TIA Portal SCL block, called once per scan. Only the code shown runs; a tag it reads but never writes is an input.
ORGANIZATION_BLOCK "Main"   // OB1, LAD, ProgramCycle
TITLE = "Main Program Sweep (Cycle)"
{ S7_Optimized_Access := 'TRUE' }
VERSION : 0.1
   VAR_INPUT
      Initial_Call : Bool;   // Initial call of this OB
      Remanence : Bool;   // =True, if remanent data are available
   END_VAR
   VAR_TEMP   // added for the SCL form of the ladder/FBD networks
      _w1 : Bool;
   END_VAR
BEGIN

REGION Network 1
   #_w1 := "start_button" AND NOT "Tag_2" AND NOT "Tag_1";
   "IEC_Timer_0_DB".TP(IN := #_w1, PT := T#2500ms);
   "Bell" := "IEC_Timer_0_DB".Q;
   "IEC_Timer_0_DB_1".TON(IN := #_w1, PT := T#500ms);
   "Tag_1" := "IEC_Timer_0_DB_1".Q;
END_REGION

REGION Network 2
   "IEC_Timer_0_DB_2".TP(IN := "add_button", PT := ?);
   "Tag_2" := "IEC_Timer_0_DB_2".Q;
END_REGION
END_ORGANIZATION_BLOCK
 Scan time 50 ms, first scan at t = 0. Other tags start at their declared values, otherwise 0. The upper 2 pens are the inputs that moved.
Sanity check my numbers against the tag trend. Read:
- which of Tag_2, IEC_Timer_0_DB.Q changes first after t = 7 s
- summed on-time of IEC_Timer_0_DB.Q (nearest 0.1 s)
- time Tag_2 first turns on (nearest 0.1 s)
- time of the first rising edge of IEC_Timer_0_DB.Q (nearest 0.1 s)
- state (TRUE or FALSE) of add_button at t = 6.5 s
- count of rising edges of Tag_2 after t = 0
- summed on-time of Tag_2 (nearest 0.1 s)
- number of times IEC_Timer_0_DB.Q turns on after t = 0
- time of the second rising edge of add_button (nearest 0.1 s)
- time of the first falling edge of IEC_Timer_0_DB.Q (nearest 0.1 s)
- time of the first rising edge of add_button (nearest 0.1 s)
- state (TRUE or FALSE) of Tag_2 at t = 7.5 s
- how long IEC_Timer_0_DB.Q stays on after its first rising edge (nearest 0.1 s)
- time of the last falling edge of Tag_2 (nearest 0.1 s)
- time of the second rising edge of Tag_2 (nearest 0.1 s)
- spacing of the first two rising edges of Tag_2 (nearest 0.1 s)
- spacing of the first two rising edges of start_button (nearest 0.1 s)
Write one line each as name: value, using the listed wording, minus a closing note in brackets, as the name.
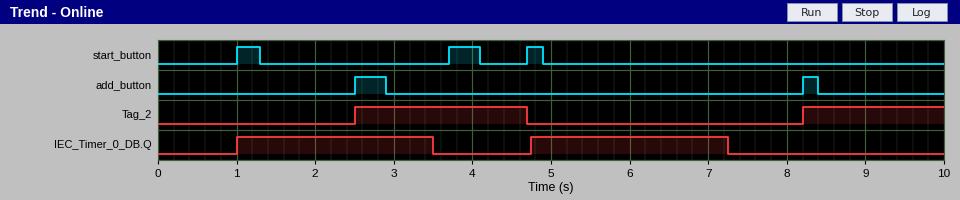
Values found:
which of Tag_2, IEC_Timer_0_DB.Q changes first after t = 7 s: IEC_Timer_0_DB.Q
summed on-time of IEC_Timer_0_DB.Q: 5.0 s
time Tag_2 first turns on: 2.5 s
time of the first rising edge of IEC_Timer_0_DB.Q: 1.0 s
state (TRUE or FALSE) of add_button at t = 6.5 s: FALSE
count of rising edges of Tag_2 after t = 0: 2
summed on-time of Tag_2: 4.0 s
number of times IEC_Timer_0_DB.Q turns on after t = 0: 2
time of the second rising edge of add_button: 8.2 s
time of the first falling edge of IEC_Timer_0_DB.Q: 3.5 s
time of the first rising edge of add_button: 2.5 s
state (TRUE or FALSE) of Tag_2 at t = 7.5 s: FALSE
how long IEC_Timer_0_DB.Q stays on after its first rising edge: 2.5 s
time of the last falling edge of Tag_2: 4.7 s
time of the second rising edge of Tag_2: 8.2 s
spacing of the first two rising edges of Tag_2: 5.7 s
spacing of the first two rising edges of start_button: 2.7 s
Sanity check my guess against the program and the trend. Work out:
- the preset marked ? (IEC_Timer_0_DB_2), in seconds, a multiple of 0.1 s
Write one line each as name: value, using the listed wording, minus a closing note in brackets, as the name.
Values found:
the preset marked ? (IEC_Timer_0_DB_2), in seconds, a multiple of 0.1 s: 2.2 s
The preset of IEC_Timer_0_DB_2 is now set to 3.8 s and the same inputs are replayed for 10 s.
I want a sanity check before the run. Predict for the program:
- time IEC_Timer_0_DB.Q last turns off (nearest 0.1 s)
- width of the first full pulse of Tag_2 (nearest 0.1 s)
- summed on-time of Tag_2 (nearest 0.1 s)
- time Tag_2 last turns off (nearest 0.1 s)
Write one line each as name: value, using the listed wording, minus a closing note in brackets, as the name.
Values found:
time IEC_Timer_0_DB.Q last turns off: 3.5 s
width of the first full pulse of Tag_2: 3.8 s
summed on-time of Tag_2: 5.6 s
time Tag_2 last turns off: 6.3 s
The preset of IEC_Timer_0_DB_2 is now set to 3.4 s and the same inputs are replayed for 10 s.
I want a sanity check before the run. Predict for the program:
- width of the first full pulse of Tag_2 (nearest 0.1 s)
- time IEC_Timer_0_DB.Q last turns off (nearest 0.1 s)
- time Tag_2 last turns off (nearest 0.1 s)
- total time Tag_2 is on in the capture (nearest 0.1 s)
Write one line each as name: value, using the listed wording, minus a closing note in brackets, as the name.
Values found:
width of the first full pulse of Tag_2: 3.4 s
time IEC_Timer_0_DB.Q last turns off: 3.5 s
time Tag_2 last turns off: 5.9 s
total time Tag_2 is on in the capture: 5.2 s
